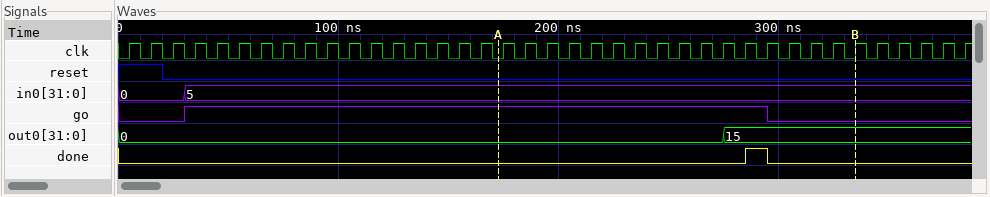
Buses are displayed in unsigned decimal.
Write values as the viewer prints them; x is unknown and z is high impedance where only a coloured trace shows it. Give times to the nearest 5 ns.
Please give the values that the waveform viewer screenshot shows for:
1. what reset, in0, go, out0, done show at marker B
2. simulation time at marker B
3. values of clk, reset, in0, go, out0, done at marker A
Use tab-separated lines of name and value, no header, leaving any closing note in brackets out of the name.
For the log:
what reset, in0, go, out0, done show at marker B	reset=0, in0=5, go=0, out0=15, done=0
simulation time at marker B	335 ns
values of clk, reset, in0, go, out0, done at marker A	clk=0, reset=0, in0=5, go=1, out0=0, done=0
